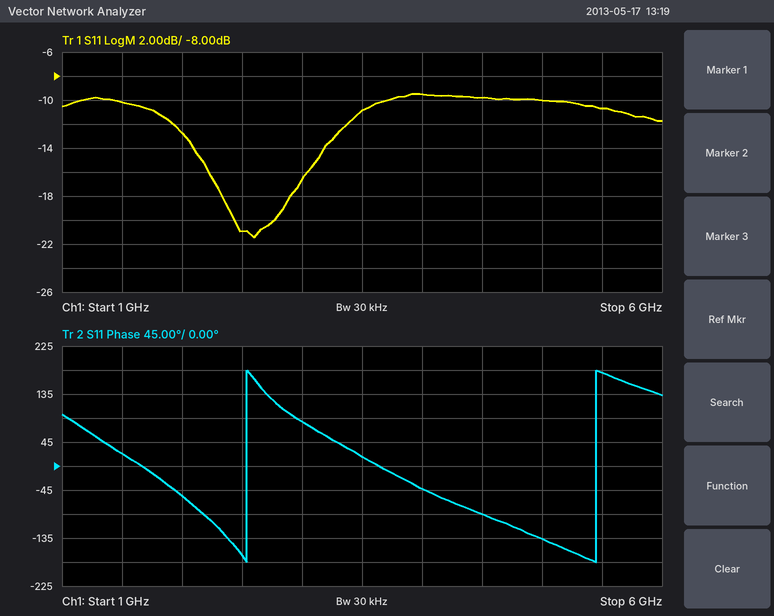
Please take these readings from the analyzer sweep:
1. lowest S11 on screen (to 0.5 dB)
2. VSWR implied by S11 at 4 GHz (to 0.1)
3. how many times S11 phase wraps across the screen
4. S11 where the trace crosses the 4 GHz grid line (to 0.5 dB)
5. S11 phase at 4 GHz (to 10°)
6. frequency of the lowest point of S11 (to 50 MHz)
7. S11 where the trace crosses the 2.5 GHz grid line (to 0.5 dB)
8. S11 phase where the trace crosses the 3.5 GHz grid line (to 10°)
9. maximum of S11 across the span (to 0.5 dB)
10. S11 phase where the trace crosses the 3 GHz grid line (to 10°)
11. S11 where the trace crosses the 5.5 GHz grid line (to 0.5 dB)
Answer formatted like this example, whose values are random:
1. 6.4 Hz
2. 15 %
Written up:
1. -21.5 dB
2. 2.0
3. 2
4. -9.5 dB
5. -40°
6. 2.60 GHz
7. -21.0 dB
8. 20°
9. -9.5 dB
10. 80°
11. -10.5 dB
